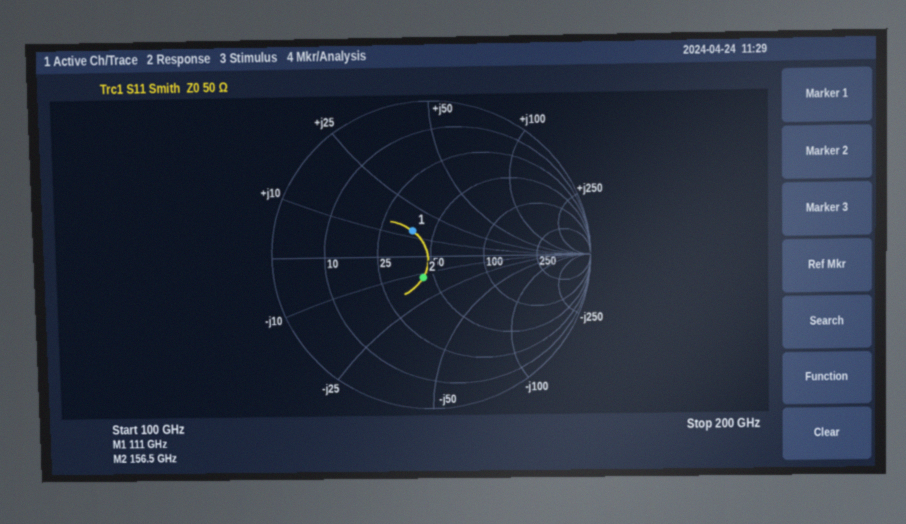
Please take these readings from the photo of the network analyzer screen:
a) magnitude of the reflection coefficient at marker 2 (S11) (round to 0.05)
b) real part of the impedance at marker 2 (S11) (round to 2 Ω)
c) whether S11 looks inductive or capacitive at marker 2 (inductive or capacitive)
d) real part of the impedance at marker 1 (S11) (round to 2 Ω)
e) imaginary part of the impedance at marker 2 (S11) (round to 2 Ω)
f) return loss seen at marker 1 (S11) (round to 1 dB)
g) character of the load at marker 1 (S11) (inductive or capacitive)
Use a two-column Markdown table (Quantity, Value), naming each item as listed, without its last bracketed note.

| Quantity | Value |
|---|---|
| magnitude of the reflection coefficient at marker 2 (S11) | 0.15 |
| real part of the impedance at marker 2 (S11) | 44 Ω |
| whether S11 looks inductive or capacitive at marker 2 | capacitive |
| real part of the impedance at marker 1 (S11) | 38 Ω |
| imaginary part of the impedance at marker 2 (S11) | -12 Ω |
| return loss seen at marker 1 (S11) | 14 dB |
| character of the load at marker 1 (S11) | inductive |
